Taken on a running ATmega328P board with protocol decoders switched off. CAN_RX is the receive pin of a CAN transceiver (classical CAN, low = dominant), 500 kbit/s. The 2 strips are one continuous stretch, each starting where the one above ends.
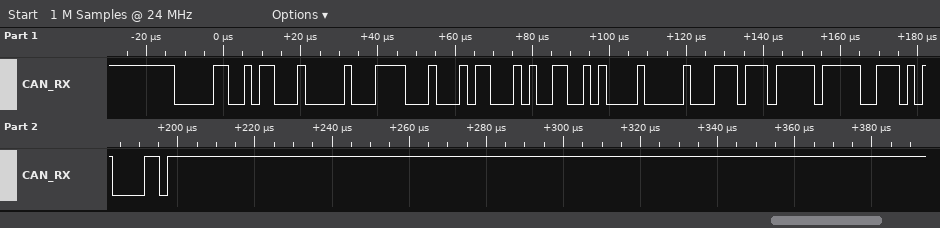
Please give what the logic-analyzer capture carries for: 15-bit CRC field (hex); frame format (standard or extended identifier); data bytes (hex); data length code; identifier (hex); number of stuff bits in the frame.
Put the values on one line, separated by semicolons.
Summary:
0x6EA1; standard; 07 88 B1 4C A1 00 EE FF; 8; 0x04B; 5
